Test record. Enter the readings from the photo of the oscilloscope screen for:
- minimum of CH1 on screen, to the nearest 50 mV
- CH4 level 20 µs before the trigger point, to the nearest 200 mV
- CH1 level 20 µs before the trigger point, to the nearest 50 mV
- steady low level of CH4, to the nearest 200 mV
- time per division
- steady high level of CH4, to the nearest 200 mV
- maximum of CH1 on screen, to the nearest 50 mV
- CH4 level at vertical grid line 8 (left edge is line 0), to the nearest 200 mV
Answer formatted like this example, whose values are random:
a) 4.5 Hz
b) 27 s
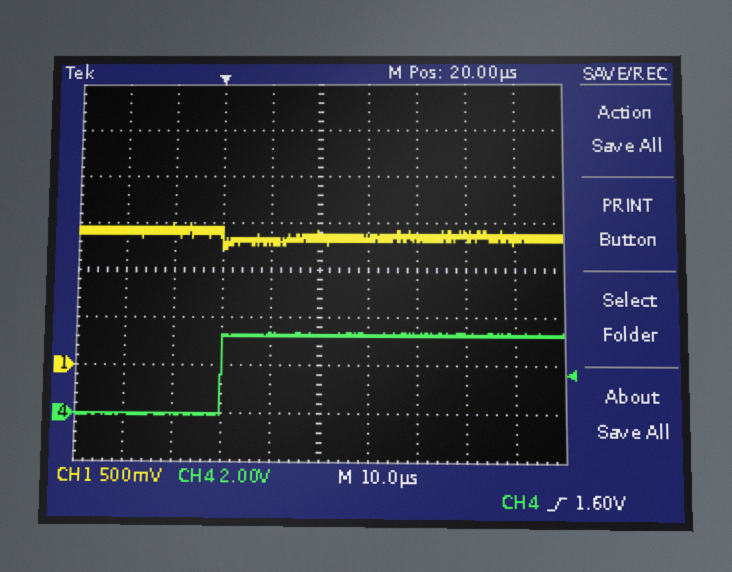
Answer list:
a) 1.20 V
b) 0.0 V
c) 1.40 V
d) 0.0 V
e) 10 µs
f) 3.2 V
g) 1.50 V
h) 3.2 V
